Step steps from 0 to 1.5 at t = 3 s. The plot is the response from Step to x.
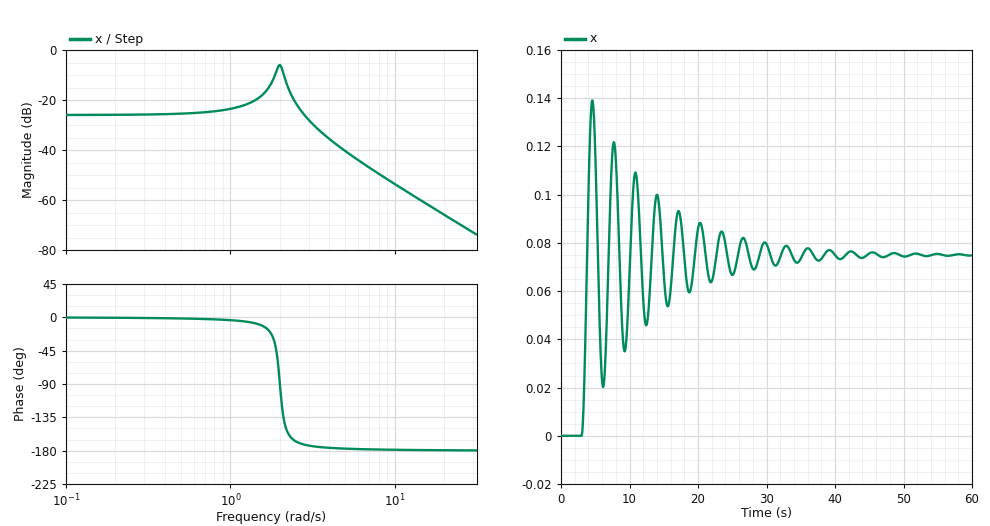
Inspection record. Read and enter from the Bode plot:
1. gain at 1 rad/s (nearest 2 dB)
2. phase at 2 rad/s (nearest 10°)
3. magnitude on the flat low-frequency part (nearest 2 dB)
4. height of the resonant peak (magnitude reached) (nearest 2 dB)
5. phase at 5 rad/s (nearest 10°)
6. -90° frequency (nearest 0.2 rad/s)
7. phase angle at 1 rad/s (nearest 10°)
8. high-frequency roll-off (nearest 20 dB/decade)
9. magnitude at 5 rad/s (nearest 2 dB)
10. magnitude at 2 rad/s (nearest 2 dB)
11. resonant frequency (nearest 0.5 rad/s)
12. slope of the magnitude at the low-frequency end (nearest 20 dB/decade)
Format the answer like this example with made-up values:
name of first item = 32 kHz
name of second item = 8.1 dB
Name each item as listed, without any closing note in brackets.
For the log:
gain at 1 rad/s = -24 dB
phase at 2 rad/s = -90°
magnitude on the flat low-frequency part = -26 dB
height of the resonant peak (magnitude reached) = -6 dB
phase at 5 rad/s = -180°
-90° frequency = 2.0 rad/s
phase angle at 1 rad/s = 0°
high-frequency roll-off = -40 dB/decade
magnitude at 5 rad/s = -40 dB
magnitude at 2 rad/s = -6 dB
resonant frequency = 2.0 rad/s
slope of the magnitude at the low-frequency end = 0 dB/decade
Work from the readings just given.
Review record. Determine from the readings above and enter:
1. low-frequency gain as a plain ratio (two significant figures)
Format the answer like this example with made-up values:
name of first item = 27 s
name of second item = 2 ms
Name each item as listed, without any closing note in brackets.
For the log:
low-frequency gain as a plain ratio = 0.050
